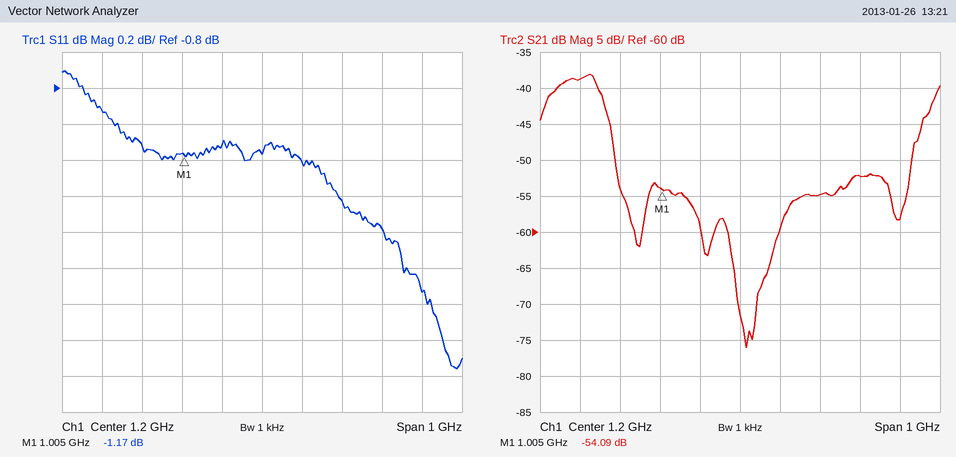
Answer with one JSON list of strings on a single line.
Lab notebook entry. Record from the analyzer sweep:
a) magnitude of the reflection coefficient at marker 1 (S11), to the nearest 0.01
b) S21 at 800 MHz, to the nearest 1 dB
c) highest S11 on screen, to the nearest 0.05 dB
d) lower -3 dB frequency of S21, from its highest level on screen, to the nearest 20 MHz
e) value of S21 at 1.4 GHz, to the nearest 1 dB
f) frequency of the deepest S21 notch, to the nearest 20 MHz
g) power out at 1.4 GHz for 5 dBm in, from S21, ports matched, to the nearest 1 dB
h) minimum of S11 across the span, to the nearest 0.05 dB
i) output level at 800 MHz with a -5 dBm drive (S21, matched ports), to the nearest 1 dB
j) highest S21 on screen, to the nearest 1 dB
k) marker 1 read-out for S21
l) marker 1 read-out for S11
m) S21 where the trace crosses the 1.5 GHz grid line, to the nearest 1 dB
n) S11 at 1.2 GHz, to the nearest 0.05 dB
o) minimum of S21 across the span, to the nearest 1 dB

["0.87", "-39 dB", "-0.70 dB", "720 MHz", "-55 dB", "1.22 GHz", "-50 dBm", "-2.35 dB", "-44 dBm", "-38 dB", "-54.09 dB", "-1.17 dB", "-52 dB", "-1.15 dB", "-76 dB"]
